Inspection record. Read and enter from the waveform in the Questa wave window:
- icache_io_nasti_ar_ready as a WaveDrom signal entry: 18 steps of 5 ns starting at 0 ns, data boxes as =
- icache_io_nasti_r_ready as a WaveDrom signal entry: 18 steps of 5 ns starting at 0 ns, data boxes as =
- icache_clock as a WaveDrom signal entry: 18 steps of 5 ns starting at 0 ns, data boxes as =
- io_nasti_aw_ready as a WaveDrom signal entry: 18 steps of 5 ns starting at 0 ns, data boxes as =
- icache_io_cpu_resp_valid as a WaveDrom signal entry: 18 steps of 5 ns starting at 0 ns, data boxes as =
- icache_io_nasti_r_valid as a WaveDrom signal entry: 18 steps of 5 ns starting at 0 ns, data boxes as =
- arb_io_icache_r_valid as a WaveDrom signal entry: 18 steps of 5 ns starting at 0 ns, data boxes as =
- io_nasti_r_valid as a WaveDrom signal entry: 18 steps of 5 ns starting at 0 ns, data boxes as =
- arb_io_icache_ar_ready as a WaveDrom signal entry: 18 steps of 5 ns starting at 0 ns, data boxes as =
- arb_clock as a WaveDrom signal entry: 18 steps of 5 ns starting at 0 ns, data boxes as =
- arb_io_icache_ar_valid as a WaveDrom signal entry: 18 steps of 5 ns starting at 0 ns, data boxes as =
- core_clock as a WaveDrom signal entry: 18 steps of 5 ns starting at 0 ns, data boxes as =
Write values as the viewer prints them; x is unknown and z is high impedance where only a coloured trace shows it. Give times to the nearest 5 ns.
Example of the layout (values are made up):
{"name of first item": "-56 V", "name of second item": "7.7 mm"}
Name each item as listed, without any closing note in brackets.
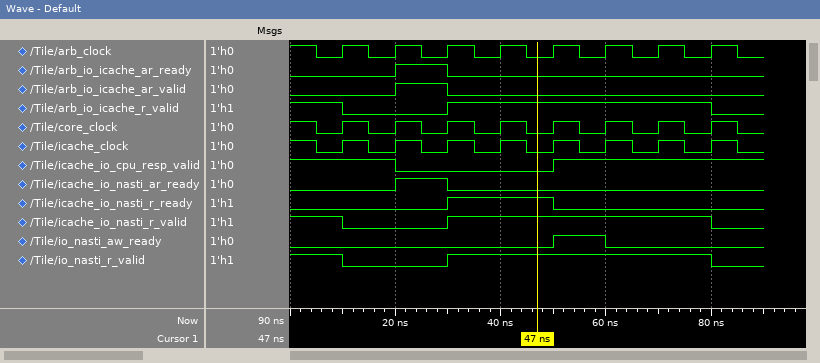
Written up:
{"icache_io_nasti_ar_ready as a WaveDrom signal entry: 18 steps of 5 ns starting at 0 ns, data boxes as =": "{name: 'icache_io_nasti_ar_ready', wave: '0...1.0...........'}", "icache_io_nasti_r_ready as a WaveDrom signal entry: 18 steps of 5 ns starting at 0 ns, data boxes as =": "{name: 'icache_io_nasti_r_ready', wave: '0.....1...0.......'}", "icache_clock as a WaveDrom signal entry: 18 steps of 5 ns starting at 0 ns, data boxes as =": "{name: 'icache_clock', wave: '101010101010101010'}", "io_nasti_aw_ready as a WaveDrom signal entry: 18 steps of 5 ns starting at 0 ns, data boxes as =": "{name: 'io_nasti_aw_ready', wave: '0.........1.0.....'}", "icache_io_cpu_resp_valid as a WaveDrom signal entry: 18 steps of 5 ns starting at 0 ns, data boxes as =": "{name: 'icache_io_cpu_resp_valid', wave: '1...0.....1.......'}", "icache_io_nasti_r_valid as a WaveDrom signal entry: 18 steps of 5 ns starting at 0 ns, data boxes as =": "{name: 'icache_io_nasti_r_valid', wave: '1.0...1.........0.'}", "arb_io_icache_r_valid as a WaveDrom signal entry: 18 steps of 5 ns starting at 0 ns, data boxes as =": "{name: 'arb_io_icache_r_valid', wave: '1.0...1.........0.'}", "io_nasti_r_valid as a WaveDrom signal entry: 18 steps of 5 ns starting at 0 ns, data boxes as =": "{name: 'io_nasti_r_valid', wave: '1.0...1.........0.'}", "arb_io_icache_ar_ready as a WaveDrom signal entry: 18 steps of 5 ns starting at 0 ns, data boxes as =": "{name: 'arb_io_icache_ar_ready', wave: '0...1.0...........'}", "arb_clock as a WaveDrom signal entry: 18 steps of 5 ns starting at 0 ns, data boxes as =": "{name: 'arb_clock', wave: '101010101010101010'}", "arb_io_icache_ar_valid as a WaveDrom signal entry: 18 steps of 5 ns starting at 0 ns, data boxes as =": "{name: 'arb_io_icache_ar_valid', wave: '0...1.0...........'}", "core_clock as a WaveDrom signal entry: 18 steps of 5 ns starting at 0 ns, data boxes as =": "{name: 'core_clock', wave: '101010101010101010'}"}
